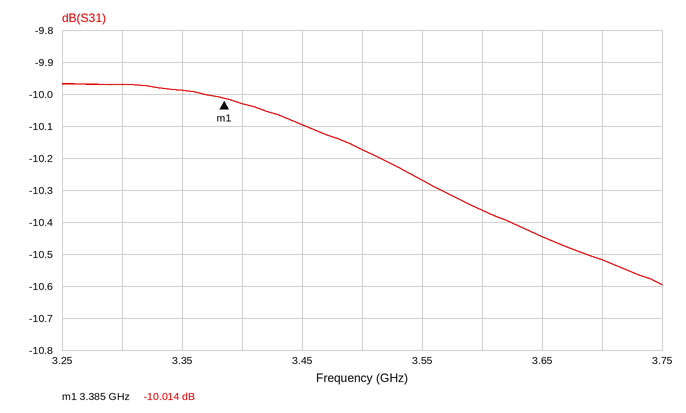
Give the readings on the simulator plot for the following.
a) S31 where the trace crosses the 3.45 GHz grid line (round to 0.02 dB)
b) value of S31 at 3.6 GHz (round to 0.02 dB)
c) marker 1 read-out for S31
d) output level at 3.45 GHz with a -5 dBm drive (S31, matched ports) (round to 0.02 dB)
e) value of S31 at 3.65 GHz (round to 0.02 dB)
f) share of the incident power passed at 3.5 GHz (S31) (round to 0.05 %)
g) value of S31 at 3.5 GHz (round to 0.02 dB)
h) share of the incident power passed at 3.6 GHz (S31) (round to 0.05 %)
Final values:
-10.10 dB
-10.36 dB
-10.014 dB
-15.10 dBm
-10.44 dB
9.60 %
-10.18 dB
9.20 %
